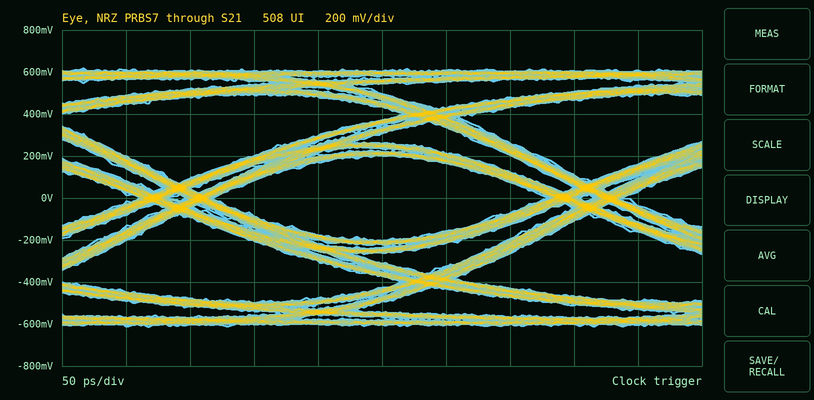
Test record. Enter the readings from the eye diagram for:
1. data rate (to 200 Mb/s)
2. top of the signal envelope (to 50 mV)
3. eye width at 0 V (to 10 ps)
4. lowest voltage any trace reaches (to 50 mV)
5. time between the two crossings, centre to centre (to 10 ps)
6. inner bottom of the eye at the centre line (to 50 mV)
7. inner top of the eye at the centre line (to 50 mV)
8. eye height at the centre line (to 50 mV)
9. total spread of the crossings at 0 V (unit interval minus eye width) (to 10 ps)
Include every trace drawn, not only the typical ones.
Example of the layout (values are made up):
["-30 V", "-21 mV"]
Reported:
["3.2 Gb/s", "600 mV", "260 ps", "-600 mV", "320 ps", "-200 mV", "200 mV", "400 mV", "60 ps"]
